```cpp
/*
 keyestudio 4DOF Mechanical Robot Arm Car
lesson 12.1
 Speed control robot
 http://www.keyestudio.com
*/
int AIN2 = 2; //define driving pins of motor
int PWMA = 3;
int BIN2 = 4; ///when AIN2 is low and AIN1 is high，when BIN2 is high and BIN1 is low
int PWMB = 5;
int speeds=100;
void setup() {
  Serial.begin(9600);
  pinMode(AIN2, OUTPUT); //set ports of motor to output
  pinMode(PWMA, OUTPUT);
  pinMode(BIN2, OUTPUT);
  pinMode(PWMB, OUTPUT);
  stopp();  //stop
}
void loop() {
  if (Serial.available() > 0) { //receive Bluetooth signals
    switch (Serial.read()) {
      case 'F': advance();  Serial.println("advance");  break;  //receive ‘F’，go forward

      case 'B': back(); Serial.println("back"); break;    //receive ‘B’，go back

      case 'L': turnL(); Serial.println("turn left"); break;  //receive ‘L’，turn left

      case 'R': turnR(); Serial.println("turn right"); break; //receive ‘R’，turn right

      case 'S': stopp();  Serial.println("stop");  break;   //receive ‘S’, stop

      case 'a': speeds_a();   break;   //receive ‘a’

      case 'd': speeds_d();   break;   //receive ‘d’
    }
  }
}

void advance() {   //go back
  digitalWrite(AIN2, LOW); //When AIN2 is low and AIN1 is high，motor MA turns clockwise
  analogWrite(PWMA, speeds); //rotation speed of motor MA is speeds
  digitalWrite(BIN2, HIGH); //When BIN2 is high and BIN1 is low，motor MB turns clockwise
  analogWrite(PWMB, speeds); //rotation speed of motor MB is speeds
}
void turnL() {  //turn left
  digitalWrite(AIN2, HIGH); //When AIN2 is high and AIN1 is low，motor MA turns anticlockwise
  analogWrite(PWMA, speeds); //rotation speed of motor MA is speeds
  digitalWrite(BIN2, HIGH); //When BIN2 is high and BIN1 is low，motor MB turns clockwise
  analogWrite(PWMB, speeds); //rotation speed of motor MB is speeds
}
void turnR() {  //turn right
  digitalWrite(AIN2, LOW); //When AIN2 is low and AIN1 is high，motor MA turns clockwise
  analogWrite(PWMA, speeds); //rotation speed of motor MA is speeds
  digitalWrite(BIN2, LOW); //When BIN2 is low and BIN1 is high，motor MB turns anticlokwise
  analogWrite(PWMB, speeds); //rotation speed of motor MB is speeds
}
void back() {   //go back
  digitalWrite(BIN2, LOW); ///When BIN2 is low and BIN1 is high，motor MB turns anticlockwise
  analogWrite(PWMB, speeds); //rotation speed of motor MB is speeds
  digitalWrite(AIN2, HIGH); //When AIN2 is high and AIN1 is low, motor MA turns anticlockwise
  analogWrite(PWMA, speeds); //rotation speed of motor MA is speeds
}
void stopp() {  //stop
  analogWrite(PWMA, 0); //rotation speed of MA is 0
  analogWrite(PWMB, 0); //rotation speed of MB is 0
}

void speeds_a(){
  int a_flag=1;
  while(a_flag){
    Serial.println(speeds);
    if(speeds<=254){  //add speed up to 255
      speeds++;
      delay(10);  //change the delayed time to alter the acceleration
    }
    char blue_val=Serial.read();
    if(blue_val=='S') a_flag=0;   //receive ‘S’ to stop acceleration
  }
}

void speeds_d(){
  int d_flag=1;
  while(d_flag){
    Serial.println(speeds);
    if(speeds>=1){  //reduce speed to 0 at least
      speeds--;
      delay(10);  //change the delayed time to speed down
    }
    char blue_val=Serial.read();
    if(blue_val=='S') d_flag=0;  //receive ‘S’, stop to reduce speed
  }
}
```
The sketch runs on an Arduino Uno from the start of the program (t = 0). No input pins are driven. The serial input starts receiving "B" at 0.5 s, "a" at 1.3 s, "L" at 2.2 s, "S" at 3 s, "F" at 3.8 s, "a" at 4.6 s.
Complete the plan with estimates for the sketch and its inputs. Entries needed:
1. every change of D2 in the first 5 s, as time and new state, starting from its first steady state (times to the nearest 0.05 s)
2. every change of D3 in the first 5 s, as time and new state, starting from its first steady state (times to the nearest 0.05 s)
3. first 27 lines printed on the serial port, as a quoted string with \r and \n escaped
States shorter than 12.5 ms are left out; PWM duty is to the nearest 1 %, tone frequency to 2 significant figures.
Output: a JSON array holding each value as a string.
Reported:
["0 s low; 0.5 s high; 3.8 s low", "0 s low; 0.5 s PWM 39 %; 3.8 s high", "\"back\\r\\n100\\r\\n101\\r\\n102\\r\\n103\\r\\n104\\r\\n105\\r\\n106\\r\\n107\\r\\n108\\r\\n109\\r\\n110\\r\\n111\\r\\n112\\r\\n113\\r\\n114\\r\\n115\\r\\n116\\r\\n117\\r\\n118\\r\\n119\\r\\n120\\r\\n121\\r\\n122\\r\\n123\\r\\n124\\r\\n125\\r\\n\""]
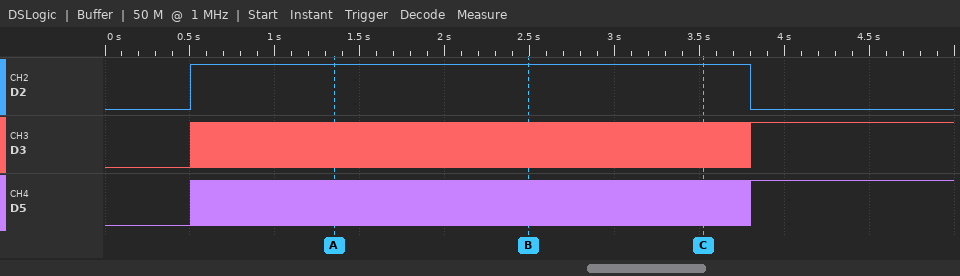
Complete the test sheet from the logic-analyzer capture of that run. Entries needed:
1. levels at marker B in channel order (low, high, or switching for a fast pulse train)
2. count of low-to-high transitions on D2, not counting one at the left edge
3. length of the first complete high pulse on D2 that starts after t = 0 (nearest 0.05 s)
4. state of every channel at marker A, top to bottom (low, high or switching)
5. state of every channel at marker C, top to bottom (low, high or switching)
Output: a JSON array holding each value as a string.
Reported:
["D2 high, D3 switching, D5 switching", "1", "3.30 s", "D2 high, D3 switching, D5 switching", "D2 high, D3 switching, D5 switching"]
